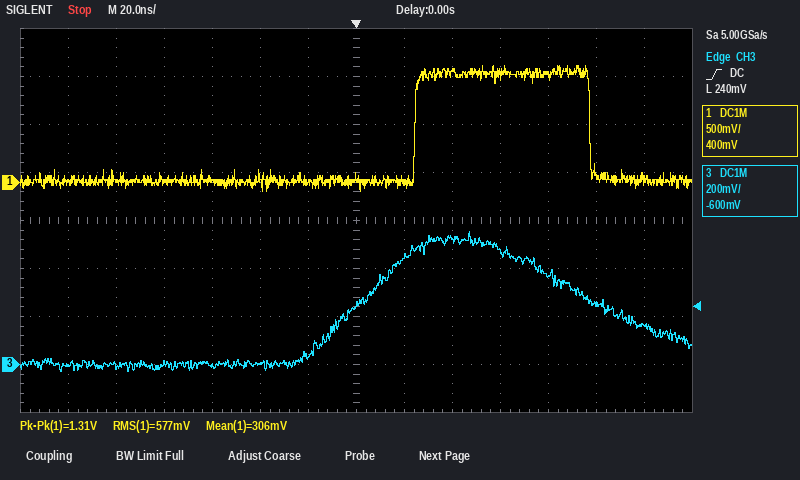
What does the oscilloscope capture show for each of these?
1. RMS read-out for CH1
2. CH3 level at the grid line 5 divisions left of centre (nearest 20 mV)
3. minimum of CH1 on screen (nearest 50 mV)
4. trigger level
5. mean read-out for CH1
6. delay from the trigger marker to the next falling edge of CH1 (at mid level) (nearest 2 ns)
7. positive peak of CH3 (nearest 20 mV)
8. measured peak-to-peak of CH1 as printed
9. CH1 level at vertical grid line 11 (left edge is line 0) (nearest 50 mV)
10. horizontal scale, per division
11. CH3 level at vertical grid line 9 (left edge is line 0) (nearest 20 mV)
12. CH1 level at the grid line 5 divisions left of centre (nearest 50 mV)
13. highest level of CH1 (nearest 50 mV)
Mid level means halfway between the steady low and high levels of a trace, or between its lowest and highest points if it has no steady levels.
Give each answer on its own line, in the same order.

577 mV
0 mV
-100 mV
240 mV
306 mV
98 ns
560 mV
1.31 V
1.10 V
20 ns
520 mV
0 mV
1.20 V
